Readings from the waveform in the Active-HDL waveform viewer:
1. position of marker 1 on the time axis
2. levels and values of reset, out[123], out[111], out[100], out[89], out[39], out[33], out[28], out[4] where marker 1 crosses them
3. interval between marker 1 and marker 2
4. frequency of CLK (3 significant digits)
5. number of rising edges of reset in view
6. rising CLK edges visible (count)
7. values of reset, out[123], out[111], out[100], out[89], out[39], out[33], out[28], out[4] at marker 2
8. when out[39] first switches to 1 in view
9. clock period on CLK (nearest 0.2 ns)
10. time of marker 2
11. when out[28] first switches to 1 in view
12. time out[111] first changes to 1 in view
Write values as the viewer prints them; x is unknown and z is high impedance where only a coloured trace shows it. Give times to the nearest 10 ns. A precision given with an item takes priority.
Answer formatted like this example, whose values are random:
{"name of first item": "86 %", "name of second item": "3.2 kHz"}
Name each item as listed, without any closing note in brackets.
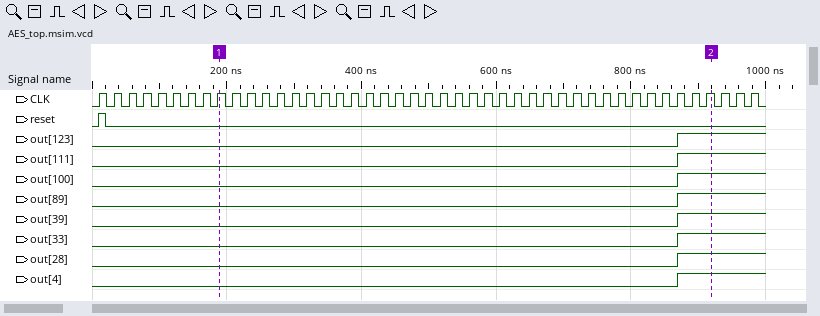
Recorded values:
{"position of marker 1 on the time axis": "190 ns", "levels and values of reset, out[123], out[111], out[100], out[89], out[39], out[33], out[28], out[4] where marker 1 crosses them": "reset=0, out[123]=0, out[111]=0, out[100]=0, out[89]=0, out[39]=0, out[33]=0, out[28]=0, out[4]=0", "interval between marker 1 and marker 2": "730 ns", "frequency of CLK": "45.5 MHz", "number of rising edges of reset in view": "1", "rising CLK edges visible": "45", "values of reset, out[123], out[111], out[100], out[89], out[39], out[33], out[28], out[4] at marker 2": "reset=0, out[123]=1, out[111]=1, out[100]=1, out[89]=1, out[39]=1, out[33]=1, out[28]=1, out[4]=1", "when out[39] first switches to 1 in view": "870 ns", "clock period on CLK": "22 ns", "time of marker 2": "920 ns", "when out[28] first switches to 1 in view": "870 ns", "time out[111] first changes to 1 in view": "870 ns"}
